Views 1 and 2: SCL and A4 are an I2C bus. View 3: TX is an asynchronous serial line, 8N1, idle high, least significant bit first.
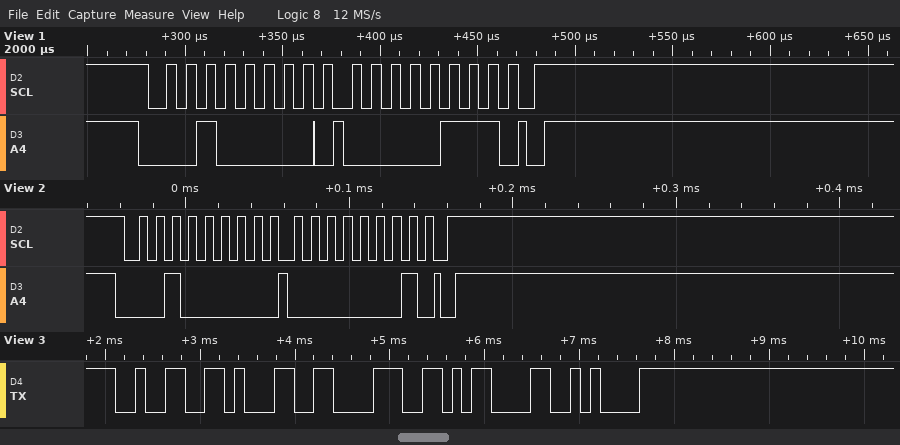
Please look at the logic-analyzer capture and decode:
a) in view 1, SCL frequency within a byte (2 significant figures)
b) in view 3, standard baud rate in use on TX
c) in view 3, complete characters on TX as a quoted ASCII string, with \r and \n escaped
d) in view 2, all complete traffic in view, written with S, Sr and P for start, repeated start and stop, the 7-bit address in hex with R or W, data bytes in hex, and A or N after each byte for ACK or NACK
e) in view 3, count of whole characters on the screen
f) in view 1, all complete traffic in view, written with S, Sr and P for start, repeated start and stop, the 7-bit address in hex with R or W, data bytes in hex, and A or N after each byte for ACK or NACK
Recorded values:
100 kHz
9600 baud
"218\r\n"
S 10W A 01 A P
5
S 10W A 07 A P
